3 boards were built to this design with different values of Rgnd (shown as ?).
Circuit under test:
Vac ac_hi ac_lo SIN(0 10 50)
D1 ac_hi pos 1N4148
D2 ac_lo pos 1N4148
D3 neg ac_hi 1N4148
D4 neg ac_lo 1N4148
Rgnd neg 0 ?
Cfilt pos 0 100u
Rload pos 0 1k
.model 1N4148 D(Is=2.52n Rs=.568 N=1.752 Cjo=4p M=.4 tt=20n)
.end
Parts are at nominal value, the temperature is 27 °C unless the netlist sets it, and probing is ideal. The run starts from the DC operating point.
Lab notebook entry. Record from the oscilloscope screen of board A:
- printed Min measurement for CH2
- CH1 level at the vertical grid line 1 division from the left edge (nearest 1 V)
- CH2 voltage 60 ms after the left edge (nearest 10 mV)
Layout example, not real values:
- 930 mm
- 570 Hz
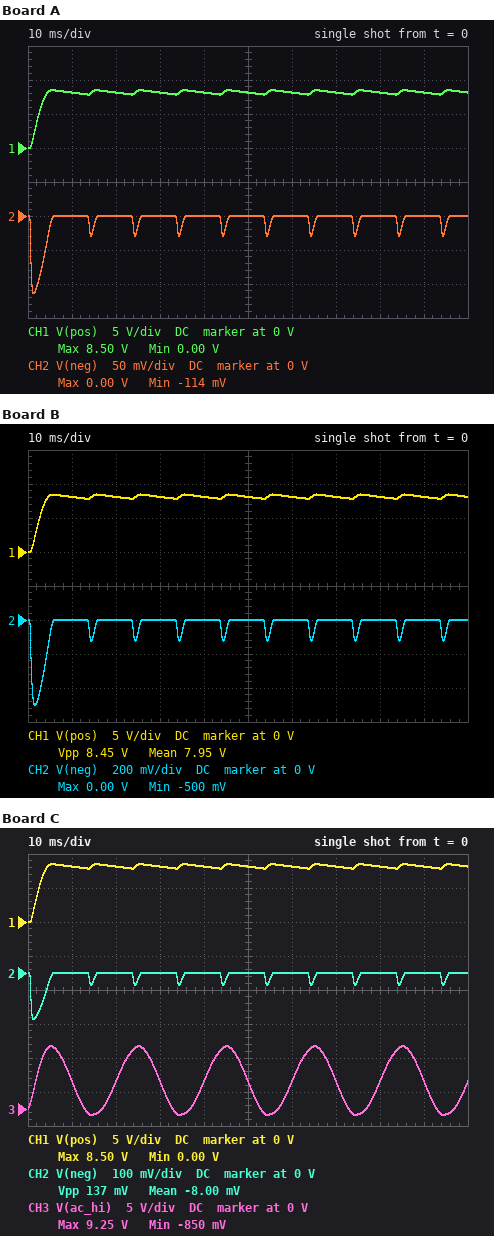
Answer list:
- -114 mV
- 8 V
- 0 V
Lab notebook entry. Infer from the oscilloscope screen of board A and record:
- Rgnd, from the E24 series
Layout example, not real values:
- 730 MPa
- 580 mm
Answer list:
- 0.39 Ω
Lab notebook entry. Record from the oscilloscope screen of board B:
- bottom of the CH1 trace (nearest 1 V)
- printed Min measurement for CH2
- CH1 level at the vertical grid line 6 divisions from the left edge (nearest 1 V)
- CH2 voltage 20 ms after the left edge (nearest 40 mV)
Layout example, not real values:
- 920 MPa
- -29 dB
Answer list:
- 0 V
- -500 mV
- 8 V
- 0 V
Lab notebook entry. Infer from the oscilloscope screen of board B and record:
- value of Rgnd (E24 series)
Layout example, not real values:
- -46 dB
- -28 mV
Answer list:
- 1.8 Ω
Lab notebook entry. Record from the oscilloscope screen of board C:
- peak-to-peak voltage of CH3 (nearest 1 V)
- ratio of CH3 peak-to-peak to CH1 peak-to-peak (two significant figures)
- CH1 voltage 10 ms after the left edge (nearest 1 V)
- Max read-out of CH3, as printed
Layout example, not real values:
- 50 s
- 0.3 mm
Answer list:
- 10 V
- 1.2
- 8 V
- 9.25 V
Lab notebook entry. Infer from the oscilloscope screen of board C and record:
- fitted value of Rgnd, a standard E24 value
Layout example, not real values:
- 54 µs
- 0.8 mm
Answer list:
- 0.47 Ω
